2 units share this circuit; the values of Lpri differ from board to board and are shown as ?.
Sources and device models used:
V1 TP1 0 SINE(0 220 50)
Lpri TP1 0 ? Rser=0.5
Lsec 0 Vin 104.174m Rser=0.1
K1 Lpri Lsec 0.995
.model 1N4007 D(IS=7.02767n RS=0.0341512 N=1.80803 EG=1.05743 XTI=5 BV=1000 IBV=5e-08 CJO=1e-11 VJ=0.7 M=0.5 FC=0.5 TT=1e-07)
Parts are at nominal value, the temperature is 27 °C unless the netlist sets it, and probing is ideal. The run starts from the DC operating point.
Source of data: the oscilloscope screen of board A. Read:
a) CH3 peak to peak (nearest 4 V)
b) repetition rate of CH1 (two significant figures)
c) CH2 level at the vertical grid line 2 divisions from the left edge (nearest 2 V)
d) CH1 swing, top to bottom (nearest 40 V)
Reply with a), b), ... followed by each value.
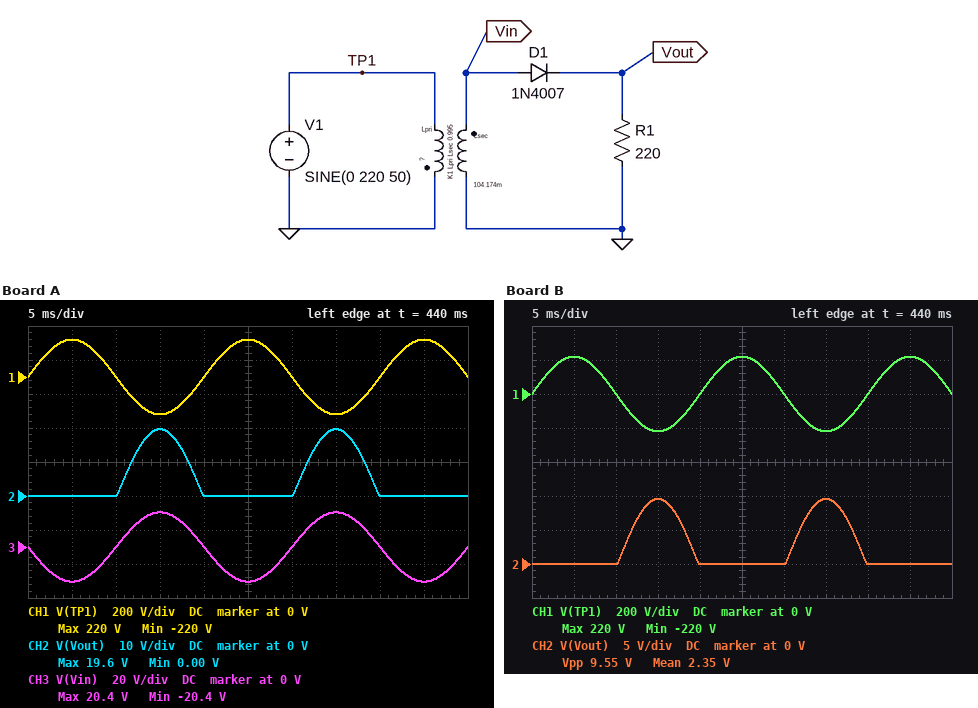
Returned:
a) 40 V
b) 50 Hz
c) 0 V
d) 440 V
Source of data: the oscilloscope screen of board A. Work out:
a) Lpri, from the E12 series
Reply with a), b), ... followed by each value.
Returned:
a) 12 H
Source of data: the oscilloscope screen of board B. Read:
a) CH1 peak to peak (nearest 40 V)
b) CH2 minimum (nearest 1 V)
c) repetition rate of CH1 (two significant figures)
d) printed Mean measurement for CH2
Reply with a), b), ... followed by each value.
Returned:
a) 440 V
b) 0 V
c) 50 Hz
d) 2.35 V
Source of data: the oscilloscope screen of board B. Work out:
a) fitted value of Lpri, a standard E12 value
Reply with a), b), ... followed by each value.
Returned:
a) 47 H
